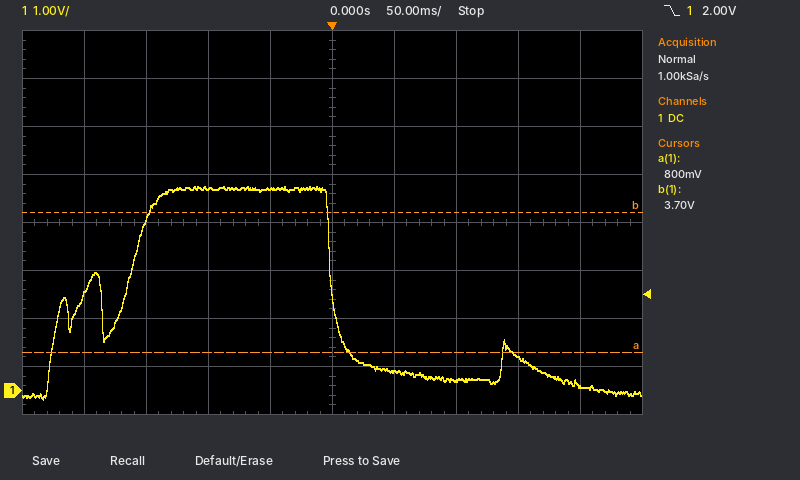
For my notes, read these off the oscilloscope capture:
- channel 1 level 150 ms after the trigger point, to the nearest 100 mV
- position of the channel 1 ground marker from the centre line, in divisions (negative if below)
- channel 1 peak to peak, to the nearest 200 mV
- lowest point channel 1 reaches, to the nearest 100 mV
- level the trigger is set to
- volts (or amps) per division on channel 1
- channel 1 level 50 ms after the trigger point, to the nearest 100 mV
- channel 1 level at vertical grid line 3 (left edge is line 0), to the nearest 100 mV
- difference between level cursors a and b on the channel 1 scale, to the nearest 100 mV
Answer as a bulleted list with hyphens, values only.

- 700 mV
- -3.5 div
- 4.4 V
- -200 mV
- 2.00 V
- 1 V
- 400 mV
- 4.2 V
- 2.9 V
